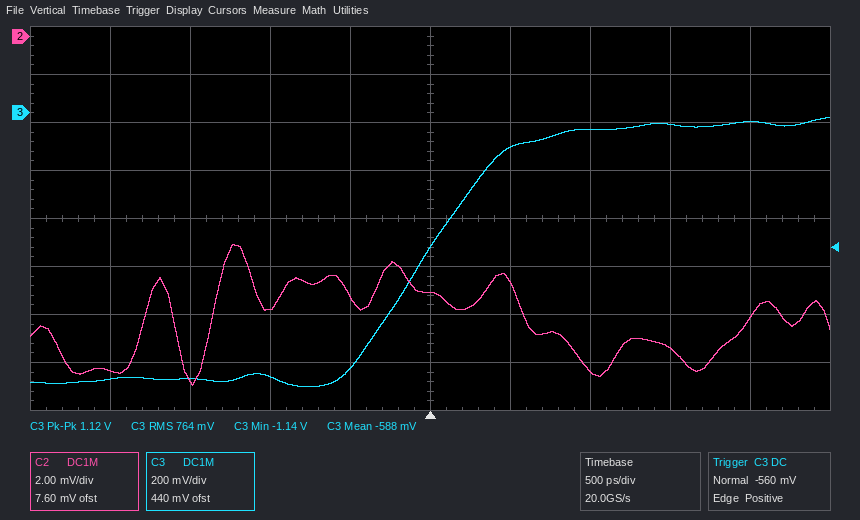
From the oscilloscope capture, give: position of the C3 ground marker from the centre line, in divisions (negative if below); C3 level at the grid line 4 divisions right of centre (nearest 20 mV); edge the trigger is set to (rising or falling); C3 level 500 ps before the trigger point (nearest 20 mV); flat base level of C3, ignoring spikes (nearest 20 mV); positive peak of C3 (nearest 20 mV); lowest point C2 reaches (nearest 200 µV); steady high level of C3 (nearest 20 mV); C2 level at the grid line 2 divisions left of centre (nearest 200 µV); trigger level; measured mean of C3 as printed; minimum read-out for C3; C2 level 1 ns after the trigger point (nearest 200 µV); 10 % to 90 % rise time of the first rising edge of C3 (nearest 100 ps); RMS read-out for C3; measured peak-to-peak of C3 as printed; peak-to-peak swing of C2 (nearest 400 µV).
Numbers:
+2.2 div
-40 mV
rising
-1.06 V
-1.12 V
-20 mV
-14.6 mV
-60 mV
-11.4 mV
-560 mV
-588 mV
-1.14 V
-14.0 mV
900 ps
764 mV
1.12 V
6.0 mV
